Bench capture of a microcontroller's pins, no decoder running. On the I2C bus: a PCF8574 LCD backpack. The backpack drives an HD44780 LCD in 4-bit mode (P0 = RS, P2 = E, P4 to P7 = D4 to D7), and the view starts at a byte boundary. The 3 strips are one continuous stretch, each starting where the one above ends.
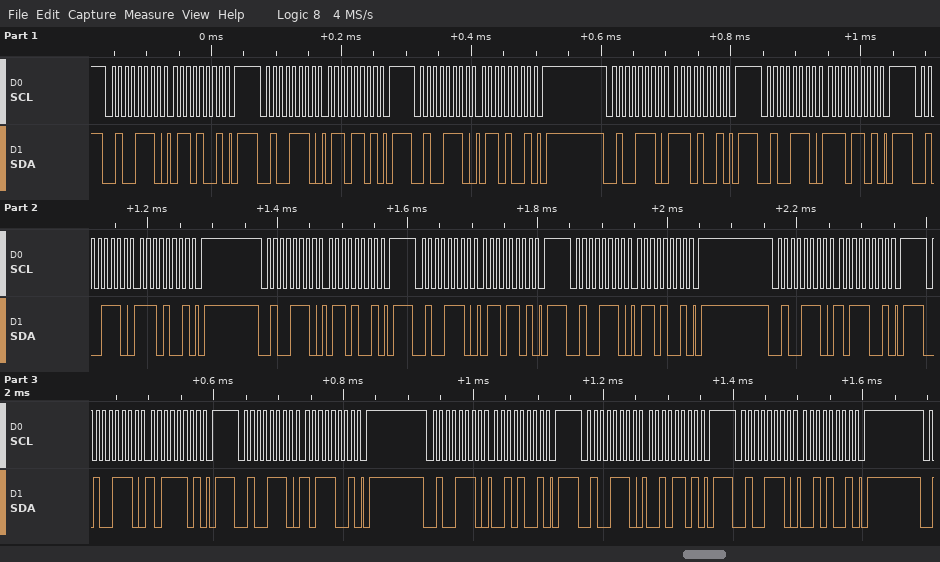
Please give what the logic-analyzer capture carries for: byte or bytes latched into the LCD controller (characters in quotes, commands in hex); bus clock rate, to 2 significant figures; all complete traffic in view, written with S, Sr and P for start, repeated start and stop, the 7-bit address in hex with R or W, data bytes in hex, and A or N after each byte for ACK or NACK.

'n' 'k'
100 kHz
S 27W A 69 A P S 27W A 6D A P S 27W A 69 A P S 27W A E9 A P S 27W A ED A P S 27W A E9 A P S 27W A 69 A P S 27W A 6D A P S 27W A 69 A P S 27W A B9 A P S 27W A BD A P S 27W A B9 A P S 27W A 29 A P S 27W A 2D A P S 27W A 29 A P
